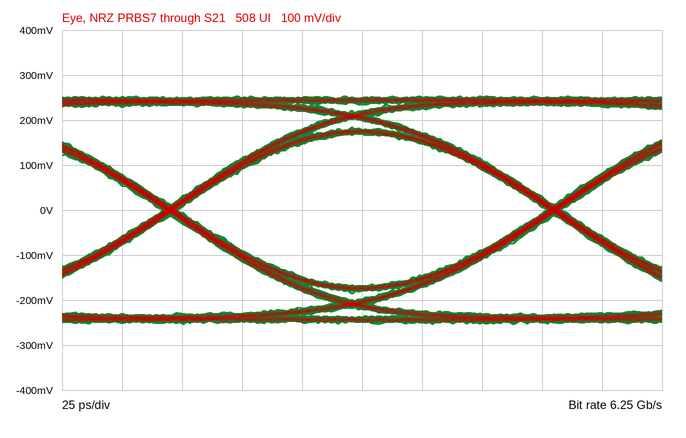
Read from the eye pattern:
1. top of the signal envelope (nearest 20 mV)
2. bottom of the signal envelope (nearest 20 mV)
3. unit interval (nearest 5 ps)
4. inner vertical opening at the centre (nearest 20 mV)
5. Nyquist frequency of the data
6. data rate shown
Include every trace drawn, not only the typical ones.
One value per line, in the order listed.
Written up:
260 mV
-260 mV
160 ps
340 mV
3.125 GHz
6.25 Gb/s
